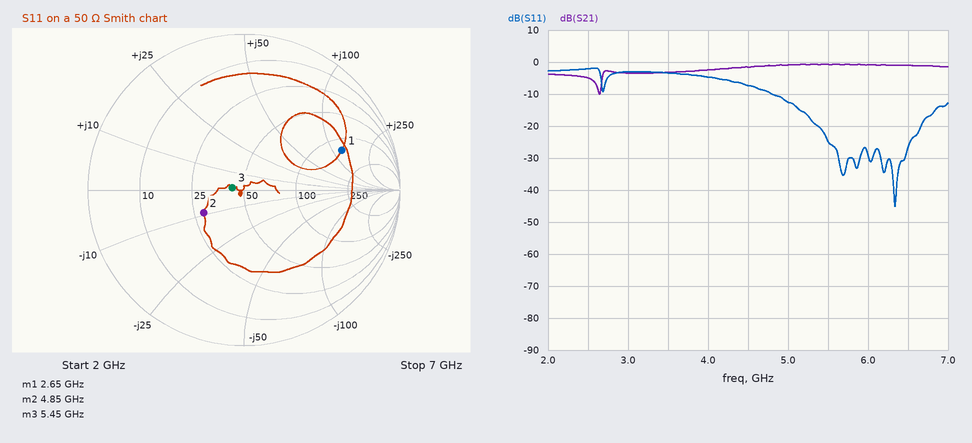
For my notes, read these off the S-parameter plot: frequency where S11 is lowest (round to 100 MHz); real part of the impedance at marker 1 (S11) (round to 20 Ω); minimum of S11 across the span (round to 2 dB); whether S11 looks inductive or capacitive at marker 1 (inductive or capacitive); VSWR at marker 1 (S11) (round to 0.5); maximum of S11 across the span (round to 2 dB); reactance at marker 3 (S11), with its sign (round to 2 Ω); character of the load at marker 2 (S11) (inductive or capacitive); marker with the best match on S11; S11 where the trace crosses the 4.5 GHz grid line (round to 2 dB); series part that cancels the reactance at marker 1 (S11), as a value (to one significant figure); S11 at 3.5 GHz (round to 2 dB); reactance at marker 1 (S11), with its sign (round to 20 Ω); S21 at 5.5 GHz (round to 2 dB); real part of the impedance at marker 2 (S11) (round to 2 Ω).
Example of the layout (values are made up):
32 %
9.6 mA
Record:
6.3 GHz
140 Ω
-46 dB
inductive
5.0
-2 dB
+2 Ω
capacitive
marker 3
-8 dB
500 fF
-4 dB
+120 Ω
0 dB
28 Ω
